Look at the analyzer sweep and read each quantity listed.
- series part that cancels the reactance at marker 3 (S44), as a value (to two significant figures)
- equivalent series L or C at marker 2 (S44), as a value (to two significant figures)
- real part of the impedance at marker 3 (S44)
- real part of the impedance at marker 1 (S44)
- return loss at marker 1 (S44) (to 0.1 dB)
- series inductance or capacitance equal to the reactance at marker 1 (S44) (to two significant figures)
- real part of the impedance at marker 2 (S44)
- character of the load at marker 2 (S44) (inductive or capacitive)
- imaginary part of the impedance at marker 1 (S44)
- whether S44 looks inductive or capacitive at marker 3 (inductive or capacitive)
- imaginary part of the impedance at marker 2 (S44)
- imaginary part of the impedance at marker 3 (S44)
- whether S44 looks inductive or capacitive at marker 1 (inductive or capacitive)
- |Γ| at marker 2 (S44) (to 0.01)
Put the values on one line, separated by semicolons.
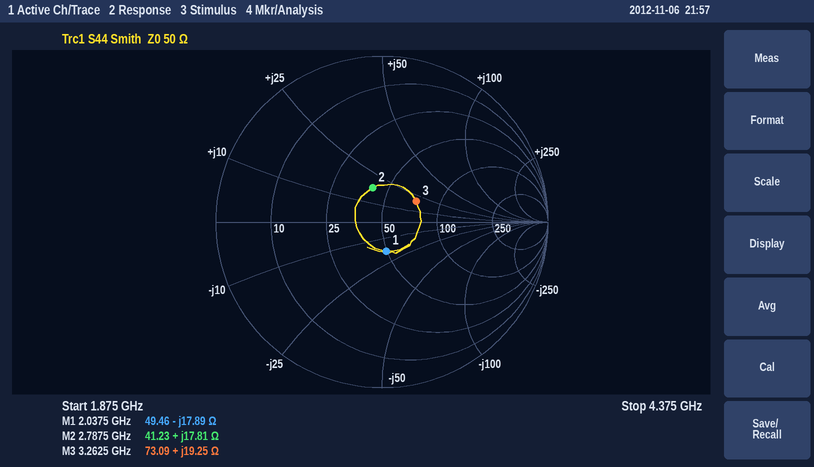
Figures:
2.5 pF; 1.0 nH; 73.09 Ω; 49.46 Ω; 15.0 dB; 4.4 pF; 41.23 Ω; inductive; -17.89 Ω; inductive; +17.81 Ω; +19.25 Ω; capacitive; 0.21
